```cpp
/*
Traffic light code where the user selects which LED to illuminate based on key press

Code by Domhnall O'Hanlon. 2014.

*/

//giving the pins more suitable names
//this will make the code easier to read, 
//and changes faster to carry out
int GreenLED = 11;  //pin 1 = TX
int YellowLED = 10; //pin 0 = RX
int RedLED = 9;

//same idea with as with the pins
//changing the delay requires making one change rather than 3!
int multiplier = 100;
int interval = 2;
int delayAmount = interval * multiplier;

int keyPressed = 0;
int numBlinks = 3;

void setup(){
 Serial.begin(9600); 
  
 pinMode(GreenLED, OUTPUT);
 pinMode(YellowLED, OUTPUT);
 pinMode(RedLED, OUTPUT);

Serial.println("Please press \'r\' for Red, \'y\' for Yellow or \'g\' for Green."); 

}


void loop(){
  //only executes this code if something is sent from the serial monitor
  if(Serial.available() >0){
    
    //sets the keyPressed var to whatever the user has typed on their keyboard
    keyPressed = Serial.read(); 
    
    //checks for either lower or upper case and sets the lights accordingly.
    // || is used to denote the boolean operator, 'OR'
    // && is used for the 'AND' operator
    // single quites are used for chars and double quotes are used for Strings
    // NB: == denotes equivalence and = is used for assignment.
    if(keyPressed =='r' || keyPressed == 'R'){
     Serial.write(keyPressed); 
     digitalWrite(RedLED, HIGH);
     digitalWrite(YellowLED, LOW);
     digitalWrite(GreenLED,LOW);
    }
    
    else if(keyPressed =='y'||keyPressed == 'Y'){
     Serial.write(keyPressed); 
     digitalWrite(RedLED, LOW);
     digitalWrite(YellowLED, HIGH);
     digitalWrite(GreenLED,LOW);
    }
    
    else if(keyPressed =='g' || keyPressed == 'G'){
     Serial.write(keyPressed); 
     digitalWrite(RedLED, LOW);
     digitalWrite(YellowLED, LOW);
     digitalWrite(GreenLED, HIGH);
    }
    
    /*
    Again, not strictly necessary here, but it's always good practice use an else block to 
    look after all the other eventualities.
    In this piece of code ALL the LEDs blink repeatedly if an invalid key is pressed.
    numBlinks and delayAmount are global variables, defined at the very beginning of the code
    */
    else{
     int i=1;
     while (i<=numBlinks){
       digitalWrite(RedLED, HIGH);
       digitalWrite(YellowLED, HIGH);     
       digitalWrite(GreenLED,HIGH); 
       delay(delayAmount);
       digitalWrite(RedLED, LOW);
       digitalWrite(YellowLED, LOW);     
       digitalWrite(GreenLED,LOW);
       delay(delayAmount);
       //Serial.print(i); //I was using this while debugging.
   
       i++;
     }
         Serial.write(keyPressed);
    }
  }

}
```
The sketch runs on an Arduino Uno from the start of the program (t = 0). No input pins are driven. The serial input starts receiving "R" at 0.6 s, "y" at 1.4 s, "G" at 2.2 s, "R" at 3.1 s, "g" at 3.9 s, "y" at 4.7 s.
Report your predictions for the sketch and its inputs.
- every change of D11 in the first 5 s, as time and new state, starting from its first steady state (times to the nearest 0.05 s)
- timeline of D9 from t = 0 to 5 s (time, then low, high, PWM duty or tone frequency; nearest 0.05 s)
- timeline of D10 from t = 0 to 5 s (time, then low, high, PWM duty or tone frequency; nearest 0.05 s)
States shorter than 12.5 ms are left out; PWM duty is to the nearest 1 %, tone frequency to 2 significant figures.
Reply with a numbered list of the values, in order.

1. 0 s low; 2.2 s high; 3.1 s low; 3.9 s high; 4.7 s low
2. 0 s low; 0.6 s high; 1.4 s low; 3.1 s high; 3.9 s low
3. 0 s low; 1.4 s high; 2.2 s low; 4.7 s high
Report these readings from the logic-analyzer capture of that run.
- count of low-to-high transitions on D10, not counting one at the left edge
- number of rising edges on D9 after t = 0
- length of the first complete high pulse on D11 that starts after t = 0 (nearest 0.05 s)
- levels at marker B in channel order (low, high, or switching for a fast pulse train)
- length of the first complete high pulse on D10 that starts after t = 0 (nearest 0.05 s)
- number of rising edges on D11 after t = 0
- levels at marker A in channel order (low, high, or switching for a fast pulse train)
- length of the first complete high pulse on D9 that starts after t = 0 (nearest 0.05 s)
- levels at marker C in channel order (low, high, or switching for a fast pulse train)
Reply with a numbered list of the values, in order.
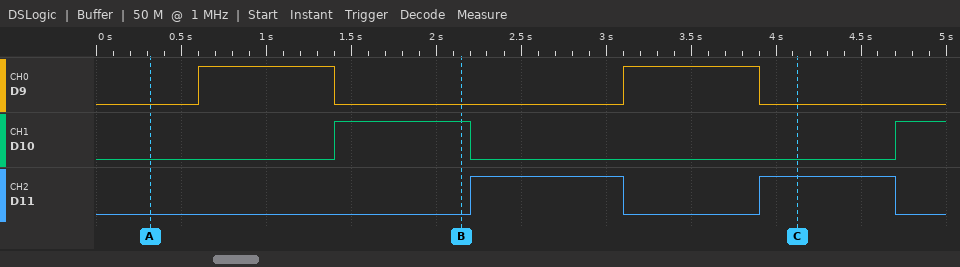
1. 2
2. 2
3. 0.90 s
4. D9 low, D10 high, D11 low
5. 0.80 s
6. 2
7. D9 low, D10 low, D11 low
8. 0.80 s
9. D9 low, D10 low, D11 high
